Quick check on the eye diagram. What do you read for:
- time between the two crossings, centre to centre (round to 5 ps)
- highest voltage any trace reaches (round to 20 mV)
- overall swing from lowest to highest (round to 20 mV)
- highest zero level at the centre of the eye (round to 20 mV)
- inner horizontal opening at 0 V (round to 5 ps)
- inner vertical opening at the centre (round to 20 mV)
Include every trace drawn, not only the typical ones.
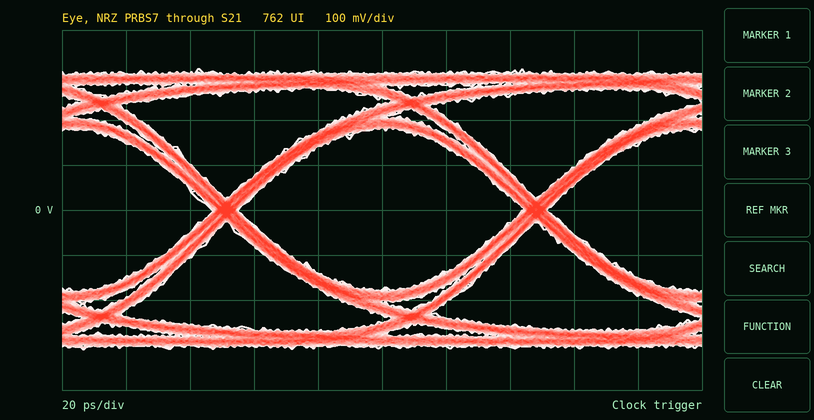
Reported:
95 ps
320 mV
620 mV
-180 mV
90 ps
360 mV
